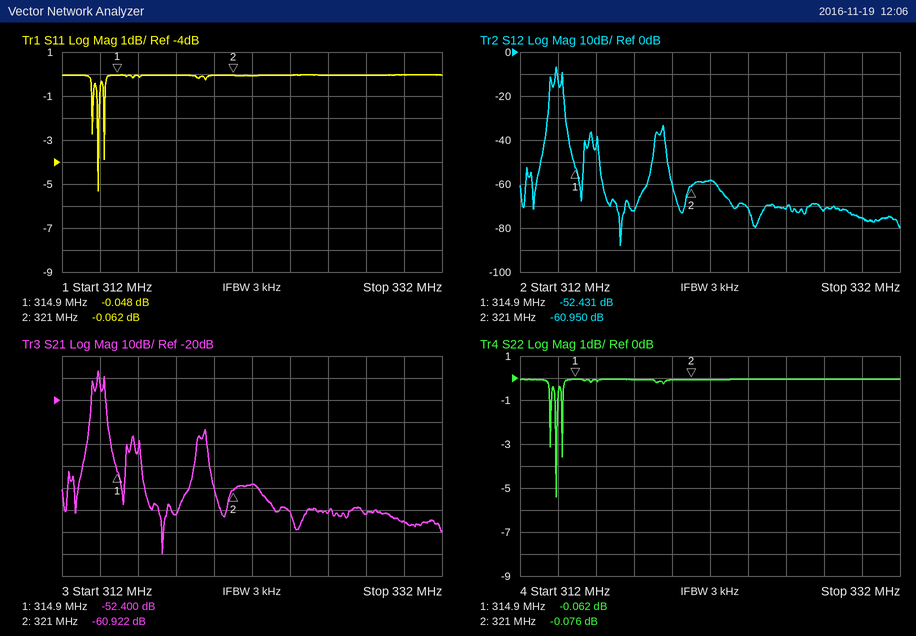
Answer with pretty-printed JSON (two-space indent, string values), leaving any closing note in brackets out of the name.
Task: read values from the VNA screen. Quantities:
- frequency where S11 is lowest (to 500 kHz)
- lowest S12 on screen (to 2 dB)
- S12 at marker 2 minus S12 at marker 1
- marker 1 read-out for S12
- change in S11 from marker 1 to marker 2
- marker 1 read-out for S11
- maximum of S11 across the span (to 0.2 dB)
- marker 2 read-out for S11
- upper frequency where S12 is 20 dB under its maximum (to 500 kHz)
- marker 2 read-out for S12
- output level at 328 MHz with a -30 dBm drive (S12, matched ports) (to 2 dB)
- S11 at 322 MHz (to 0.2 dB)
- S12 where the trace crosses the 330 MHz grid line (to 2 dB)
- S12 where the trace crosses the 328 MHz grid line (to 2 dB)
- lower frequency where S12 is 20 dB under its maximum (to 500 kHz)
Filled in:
{
  "frequency where S11 is lowest": "314.0 MHz",
  "lowest S12 on screen": "-88 dB",
  "S12 at marker 2 minus S12 at marker 1": "-8.519 dB",
  "marker 1 read-out for S12": "-52.431 dB",
  "change in S11 from marker 1 to marker 2": "-0.014 dB",
  "marker 1 read-out for S11": "-0.048 dB",
  "maximum of S11 across the span": "0.0 dB",
  "marker 2 read-out for S11": "-0.062 dB",
  "upper frequency where S12 is 20 dB under its maximum": "314.5 MHz",
  "marker 2 read-out for S12": "-60.950 dB",
  "output level at 328 MHz with a -30 dBm drive (S12, matched ports)": "-102 dBm",
  "S11 at 322 MHz": "0.0 dB",
  "S12 where the trace crosses the 330 MHz grid line": "-76 dB",
  "S12 where the trace crosses the 328 MHz grid line": "-72 dB",
  "lower frequency where S12 is 20 dB under its maximum": "313.5 MHz"
}
